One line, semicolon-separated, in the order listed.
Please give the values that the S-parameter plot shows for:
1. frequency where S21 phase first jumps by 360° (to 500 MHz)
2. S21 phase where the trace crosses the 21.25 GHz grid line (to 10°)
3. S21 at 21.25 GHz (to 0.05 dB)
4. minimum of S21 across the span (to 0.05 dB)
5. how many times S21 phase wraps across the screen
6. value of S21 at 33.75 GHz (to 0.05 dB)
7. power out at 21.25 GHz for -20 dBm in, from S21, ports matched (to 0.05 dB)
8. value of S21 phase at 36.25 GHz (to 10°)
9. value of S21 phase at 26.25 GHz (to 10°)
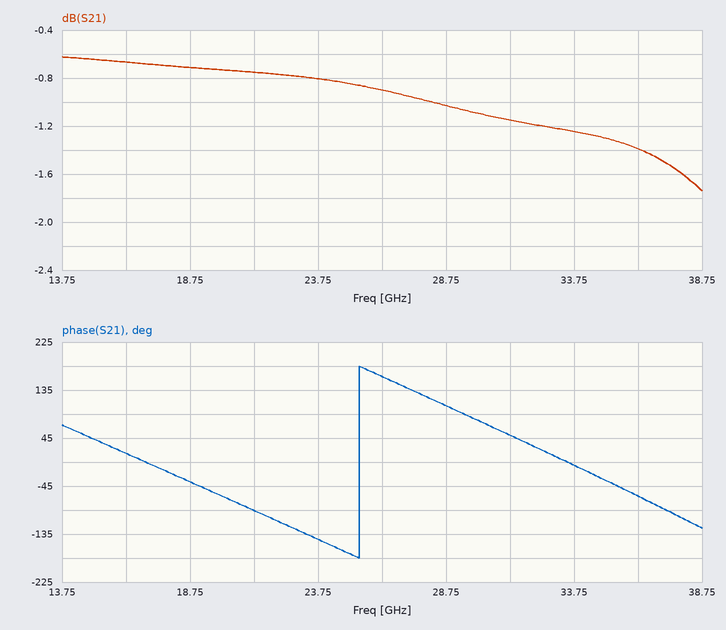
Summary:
25.5 GHz; -90°; -0.75 dB; -1.75 dB; 1; -1.25 dB; -20.75 dBm; -60°; 160°
